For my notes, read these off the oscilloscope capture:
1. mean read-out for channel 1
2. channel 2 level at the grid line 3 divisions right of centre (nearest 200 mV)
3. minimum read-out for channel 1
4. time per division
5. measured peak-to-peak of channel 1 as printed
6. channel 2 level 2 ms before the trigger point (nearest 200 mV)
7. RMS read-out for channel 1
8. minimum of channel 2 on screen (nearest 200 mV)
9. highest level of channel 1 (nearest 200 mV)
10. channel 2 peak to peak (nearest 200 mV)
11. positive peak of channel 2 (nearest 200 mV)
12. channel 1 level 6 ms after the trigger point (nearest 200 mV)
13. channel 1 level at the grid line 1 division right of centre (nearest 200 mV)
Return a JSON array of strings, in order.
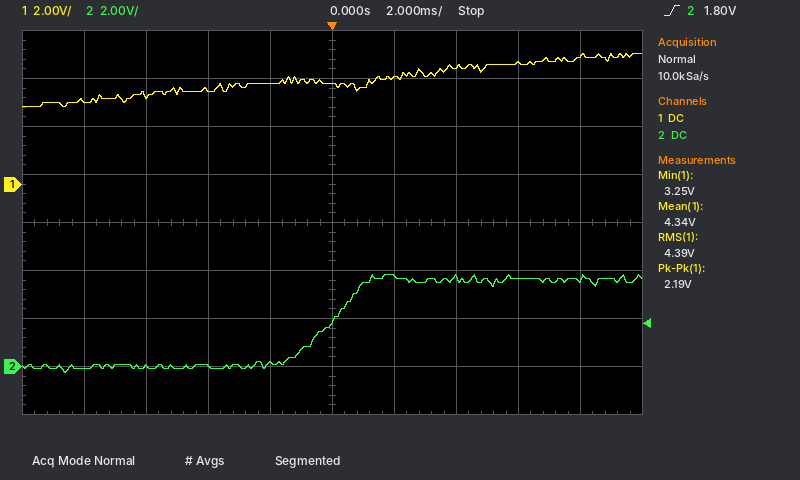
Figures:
["4.34 V", "3.6 V", "3.25 V", "2 ms", "2.19 V", "200 mV", "4.39 V", "-200 mV", "5.4 V", "4.0 V", "3.8 V", "5.0 V", "4.4 V"]
